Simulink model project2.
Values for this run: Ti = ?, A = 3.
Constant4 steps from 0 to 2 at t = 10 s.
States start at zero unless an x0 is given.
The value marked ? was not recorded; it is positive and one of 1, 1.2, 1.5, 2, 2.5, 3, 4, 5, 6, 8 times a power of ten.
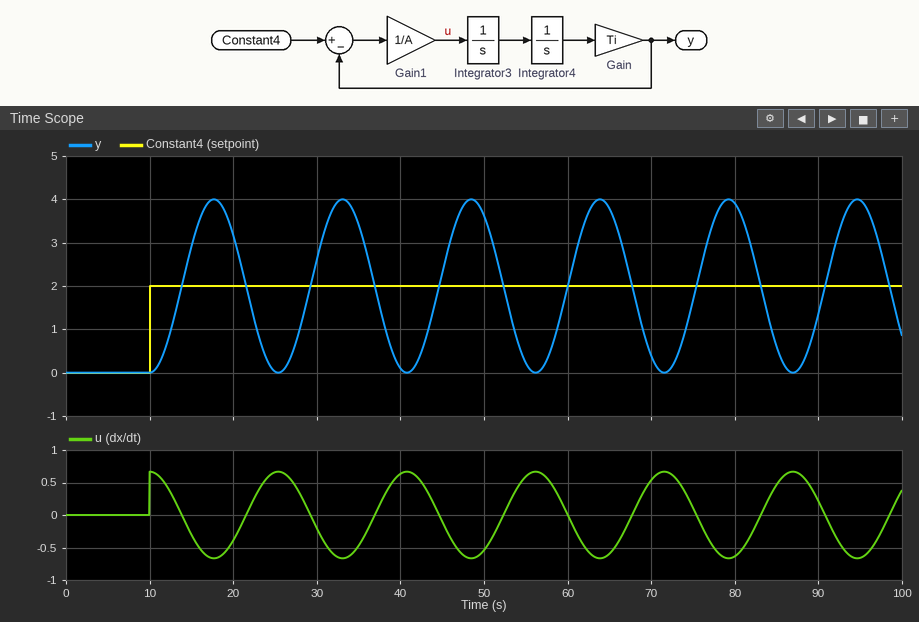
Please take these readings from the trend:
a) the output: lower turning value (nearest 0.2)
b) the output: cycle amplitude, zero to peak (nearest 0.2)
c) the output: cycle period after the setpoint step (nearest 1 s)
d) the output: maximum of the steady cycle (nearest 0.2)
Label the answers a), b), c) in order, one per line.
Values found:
a) 0.0
b) 2.0
c) 15 s
d) 4.0
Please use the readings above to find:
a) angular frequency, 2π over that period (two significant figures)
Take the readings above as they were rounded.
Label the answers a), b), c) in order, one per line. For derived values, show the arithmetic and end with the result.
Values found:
a) 2π / 15 = 0.42 rad/s
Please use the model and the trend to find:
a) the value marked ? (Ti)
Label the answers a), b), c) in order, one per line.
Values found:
a) 0.5
